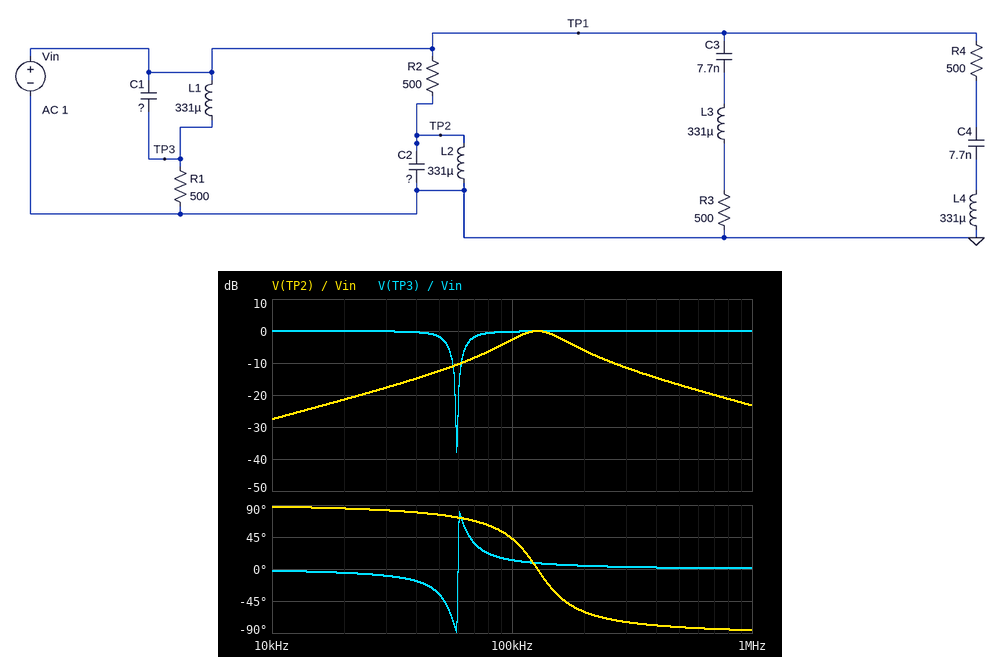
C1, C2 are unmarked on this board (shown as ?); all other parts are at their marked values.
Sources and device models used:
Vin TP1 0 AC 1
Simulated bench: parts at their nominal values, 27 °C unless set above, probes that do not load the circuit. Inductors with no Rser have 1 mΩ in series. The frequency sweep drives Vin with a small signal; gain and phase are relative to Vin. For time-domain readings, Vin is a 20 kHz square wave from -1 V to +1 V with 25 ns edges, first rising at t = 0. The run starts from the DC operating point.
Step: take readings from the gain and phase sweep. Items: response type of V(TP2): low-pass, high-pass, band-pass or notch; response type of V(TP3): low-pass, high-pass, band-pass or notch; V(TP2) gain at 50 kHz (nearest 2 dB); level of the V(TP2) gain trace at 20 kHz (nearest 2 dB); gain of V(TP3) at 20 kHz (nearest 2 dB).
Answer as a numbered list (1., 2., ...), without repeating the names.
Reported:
1. band-pass
2. notch
3. -12 dB
4. -22 dB
5. 0 dB
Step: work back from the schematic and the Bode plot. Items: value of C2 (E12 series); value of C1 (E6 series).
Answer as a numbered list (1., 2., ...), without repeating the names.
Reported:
1. 4.7 nF
2. 22 nF
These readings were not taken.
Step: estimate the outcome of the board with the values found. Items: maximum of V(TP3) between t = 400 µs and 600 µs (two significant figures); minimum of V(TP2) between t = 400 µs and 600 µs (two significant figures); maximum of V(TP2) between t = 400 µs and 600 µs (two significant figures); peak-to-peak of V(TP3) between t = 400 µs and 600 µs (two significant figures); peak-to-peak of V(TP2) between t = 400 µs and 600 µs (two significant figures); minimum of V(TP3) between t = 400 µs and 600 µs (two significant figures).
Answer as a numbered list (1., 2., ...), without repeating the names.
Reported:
1. 1.4 V
2. -740 mV
3. 740 mV
4. 2.8 V
5. 1.5 V
6. -1.4 V
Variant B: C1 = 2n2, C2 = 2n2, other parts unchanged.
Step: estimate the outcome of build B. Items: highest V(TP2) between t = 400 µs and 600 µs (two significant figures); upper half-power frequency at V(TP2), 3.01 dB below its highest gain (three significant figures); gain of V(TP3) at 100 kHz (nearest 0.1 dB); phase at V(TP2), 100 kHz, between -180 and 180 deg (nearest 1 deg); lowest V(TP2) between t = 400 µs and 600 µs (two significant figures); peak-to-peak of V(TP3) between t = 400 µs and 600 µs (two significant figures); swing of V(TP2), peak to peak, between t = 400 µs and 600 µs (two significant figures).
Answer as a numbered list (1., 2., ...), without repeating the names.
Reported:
1. 950 mV
2. 272 kHz
3. -1.3 dB
4. 60 deg
5. -950 mV
6. 2.5 V
7. 1.9 V
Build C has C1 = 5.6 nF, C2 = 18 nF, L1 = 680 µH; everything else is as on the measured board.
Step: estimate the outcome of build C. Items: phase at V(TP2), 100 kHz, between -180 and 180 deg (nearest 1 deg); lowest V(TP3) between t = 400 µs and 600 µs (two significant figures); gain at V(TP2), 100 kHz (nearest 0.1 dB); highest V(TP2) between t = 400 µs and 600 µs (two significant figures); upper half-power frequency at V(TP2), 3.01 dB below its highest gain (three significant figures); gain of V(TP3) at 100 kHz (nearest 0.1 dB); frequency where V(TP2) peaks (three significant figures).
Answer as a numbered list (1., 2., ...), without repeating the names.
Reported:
1. -73 deg
2. -1.3 V
3. -10.6 dB
4. 550 mV
5. 74.6 kHz
6. -5.9 dB
7. 65.2 kHz
